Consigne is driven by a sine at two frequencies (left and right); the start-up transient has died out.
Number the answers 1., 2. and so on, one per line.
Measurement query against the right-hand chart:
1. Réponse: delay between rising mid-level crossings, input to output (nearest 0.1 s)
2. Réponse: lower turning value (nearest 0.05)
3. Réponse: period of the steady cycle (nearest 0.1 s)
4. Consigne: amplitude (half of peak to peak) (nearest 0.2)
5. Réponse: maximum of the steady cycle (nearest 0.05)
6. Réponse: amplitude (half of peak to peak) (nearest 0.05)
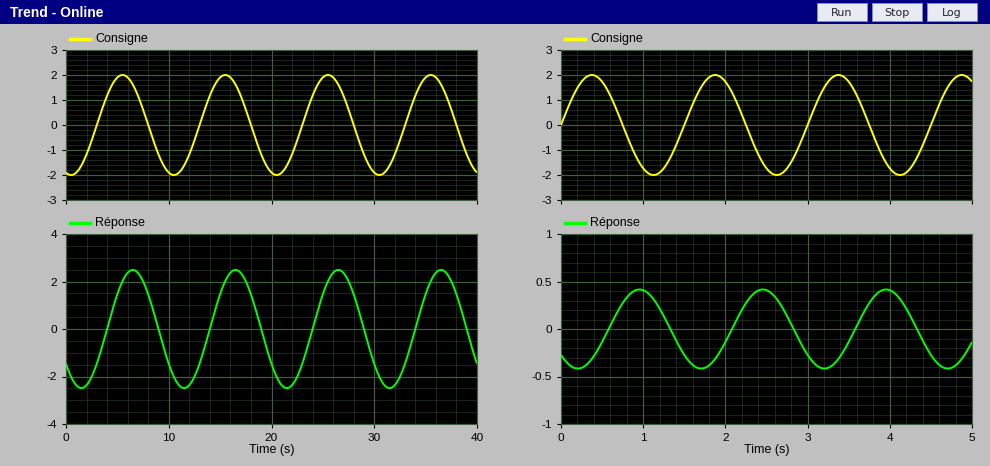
1. 0.6 s
2. -0.40
3. 1.5 s
4. 2.0
5. 0.40
6. 0.40
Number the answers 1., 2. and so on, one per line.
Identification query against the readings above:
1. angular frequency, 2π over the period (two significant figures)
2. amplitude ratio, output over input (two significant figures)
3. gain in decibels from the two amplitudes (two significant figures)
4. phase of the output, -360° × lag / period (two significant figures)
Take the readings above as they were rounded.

1. 4.2 rad/s
2. 0.20
3. -14 dB
4. -140°
